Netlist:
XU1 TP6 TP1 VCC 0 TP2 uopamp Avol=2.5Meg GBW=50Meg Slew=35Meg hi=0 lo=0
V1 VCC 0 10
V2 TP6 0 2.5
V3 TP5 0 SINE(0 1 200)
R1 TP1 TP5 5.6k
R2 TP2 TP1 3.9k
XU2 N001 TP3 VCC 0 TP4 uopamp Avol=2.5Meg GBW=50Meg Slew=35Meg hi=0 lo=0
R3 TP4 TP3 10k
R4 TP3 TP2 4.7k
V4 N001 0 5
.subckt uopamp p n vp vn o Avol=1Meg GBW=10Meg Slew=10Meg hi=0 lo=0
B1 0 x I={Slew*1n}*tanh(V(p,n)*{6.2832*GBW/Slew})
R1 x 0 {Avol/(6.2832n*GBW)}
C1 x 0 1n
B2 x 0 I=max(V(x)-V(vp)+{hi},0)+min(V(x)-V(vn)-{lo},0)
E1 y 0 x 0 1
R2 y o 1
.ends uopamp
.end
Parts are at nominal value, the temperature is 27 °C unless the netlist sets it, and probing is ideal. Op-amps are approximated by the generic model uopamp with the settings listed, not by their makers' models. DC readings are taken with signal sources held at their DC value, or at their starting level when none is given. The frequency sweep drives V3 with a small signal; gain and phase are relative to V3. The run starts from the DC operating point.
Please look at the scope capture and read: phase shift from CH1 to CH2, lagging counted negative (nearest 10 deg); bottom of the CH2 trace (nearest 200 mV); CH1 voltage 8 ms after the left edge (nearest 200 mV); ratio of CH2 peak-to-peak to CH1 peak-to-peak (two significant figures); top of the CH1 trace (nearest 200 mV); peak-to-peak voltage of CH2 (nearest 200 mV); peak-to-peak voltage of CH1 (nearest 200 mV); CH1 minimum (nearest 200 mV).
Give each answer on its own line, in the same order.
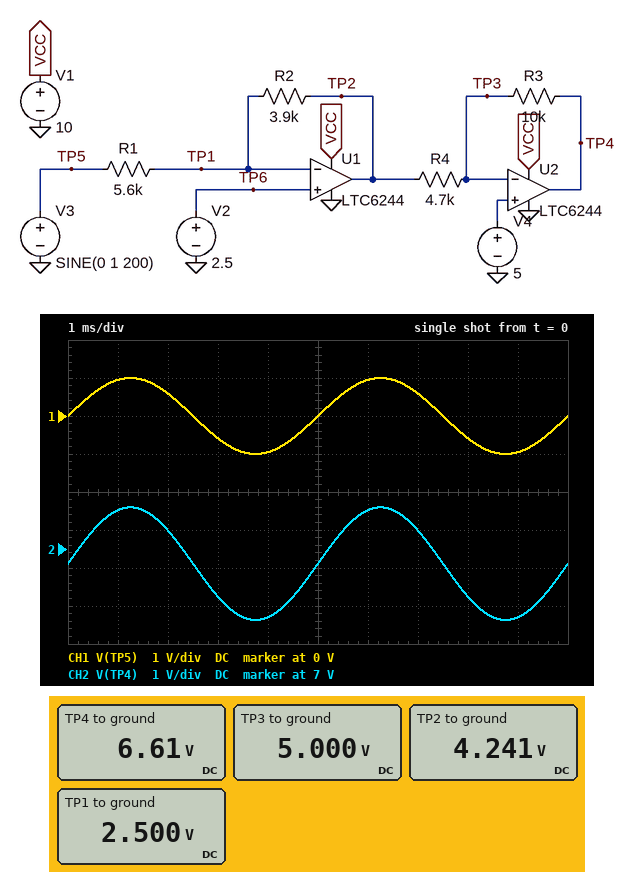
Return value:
0 deg
5.2 V
-600 mV
1.5
1.0 V
3.0 V
2.0 V
-1.0 V
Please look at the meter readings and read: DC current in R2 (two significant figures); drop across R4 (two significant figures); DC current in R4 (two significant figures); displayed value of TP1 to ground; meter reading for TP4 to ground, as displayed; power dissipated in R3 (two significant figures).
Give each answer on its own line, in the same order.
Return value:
450 µA
760 mV
160 µA
2.500 V
6.61 V
260 µW
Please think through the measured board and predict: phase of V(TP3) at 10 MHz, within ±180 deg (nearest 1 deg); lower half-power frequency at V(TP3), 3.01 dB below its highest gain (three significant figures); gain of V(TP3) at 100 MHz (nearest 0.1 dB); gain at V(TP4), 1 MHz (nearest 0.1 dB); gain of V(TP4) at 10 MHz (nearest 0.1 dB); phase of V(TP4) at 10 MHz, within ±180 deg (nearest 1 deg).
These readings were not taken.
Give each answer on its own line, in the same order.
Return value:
-141 deg
8.70 MHz
-17.6 dB
3.4 dB
1.5 dB
-51 deg
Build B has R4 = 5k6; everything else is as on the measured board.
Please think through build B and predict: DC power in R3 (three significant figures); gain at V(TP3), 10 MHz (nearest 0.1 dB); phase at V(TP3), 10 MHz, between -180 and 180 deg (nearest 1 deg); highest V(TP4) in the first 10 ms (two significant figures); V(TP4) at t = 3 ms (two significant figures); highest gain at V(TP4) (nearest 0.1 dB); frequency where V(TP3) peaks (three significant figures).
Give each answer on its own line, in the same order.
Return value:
184 µW
-13.7 dB
-138 deg
7.6 V
5.6 V
1.9 dB
23.0 MHz
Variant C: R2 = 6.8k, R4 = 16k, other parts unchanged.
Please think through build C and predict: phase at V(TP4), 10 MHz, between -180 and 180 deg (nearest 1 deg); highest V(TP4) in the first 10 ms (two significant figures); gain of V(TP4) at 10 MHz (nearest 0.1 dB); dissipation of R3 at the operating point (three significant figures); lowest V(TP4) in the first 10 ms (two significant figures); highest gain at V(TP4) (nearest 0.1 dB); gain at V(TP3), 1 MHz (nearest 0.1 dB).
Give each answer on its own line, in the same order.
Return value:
-42 deg
5.4 V
-3.6 dB
11.2 µW
3.9 V
-2.4 dB
-36.4 dB
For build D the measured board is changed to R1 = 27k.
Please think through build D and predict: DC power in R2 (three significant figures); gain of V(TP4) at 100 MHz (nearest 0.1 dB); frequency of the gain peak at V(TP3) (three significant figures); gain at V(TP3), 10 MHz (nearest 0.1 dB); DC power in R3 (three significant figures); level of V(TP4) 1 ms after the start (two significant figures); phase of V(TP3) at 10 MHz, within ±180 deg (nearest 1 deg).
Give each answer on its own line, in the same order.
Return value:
33.4 µW
-34.2 dB
26.4 MHz
-25.9 dB
2.07 mW
9.8 V
-135 deg
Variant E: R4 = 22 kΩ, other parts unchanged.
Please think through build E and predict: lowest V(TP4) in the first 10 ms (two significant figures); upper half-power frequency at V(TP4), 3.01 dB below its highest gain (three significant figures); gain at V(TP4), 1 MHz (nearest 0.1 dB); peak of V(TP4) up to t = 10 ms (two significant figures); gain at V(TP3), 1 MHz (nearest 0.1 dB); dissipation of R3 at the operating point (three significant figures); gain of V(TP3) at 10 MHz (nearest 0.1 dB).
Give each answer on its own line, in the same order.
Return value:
5.0 V
20.4 MHz
-10.0 dB
5.7 V
-44.0 dB
11.9 µW
-24.8 dB
